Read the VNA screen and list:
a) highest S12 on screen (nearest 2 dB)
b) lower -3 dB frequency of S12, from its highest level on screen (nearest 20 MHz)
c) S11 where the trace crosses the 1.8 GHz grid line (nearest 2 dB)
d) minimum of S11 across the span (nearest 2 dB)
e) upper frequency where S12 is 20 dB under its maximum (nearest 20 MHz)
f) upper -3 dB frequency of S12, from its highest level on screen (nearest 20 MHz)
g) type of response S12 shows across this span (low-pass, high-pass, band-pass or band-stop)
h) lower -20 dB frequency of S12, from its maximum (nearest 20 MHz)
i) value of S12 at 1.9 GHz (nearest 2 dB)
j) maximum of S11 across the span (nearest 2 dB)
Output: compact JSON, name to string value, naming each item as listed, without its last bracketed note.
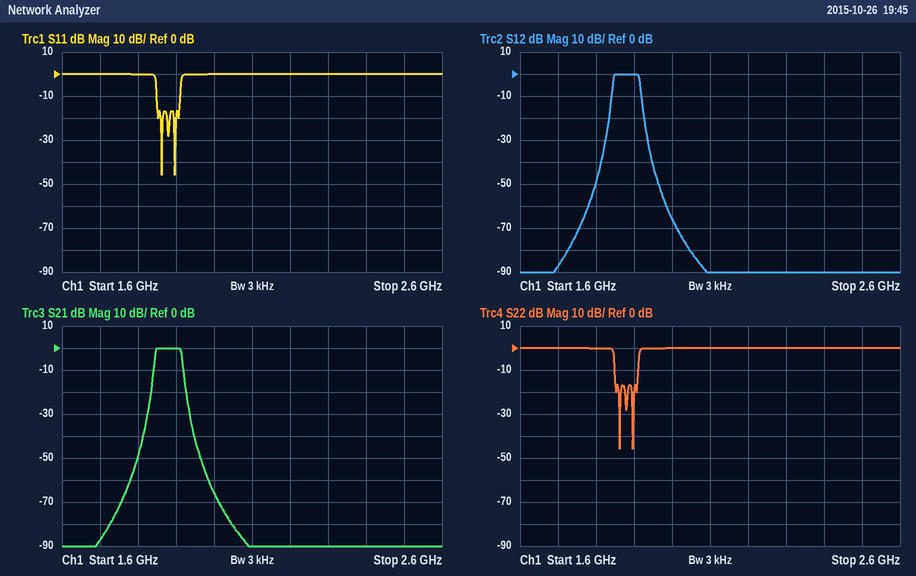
{"highest S12 on screen": "0 dB", "lower -3 dB frequency of S12, from its highest level on screen": "1.84 GHz", "S11 where the trace crosses the 1.8 GHz grid line": "0 dB", "minimum of S11 across the span": "-46 dB", "upper frequency where S12 is 20 dB under its maximum": "1.92 GHz", "upper -3 dB frequency of S12, from its highest level on screen": "1.92 GHz", "type of response S12 shows across this span": "band-pass", "lower -20 dB frequency of S12, from its maximum": "1.84 GHz", "value of S12 at 1.9 GHz": "0 dB", "maximum of S11 across the span": "0 dB"}
